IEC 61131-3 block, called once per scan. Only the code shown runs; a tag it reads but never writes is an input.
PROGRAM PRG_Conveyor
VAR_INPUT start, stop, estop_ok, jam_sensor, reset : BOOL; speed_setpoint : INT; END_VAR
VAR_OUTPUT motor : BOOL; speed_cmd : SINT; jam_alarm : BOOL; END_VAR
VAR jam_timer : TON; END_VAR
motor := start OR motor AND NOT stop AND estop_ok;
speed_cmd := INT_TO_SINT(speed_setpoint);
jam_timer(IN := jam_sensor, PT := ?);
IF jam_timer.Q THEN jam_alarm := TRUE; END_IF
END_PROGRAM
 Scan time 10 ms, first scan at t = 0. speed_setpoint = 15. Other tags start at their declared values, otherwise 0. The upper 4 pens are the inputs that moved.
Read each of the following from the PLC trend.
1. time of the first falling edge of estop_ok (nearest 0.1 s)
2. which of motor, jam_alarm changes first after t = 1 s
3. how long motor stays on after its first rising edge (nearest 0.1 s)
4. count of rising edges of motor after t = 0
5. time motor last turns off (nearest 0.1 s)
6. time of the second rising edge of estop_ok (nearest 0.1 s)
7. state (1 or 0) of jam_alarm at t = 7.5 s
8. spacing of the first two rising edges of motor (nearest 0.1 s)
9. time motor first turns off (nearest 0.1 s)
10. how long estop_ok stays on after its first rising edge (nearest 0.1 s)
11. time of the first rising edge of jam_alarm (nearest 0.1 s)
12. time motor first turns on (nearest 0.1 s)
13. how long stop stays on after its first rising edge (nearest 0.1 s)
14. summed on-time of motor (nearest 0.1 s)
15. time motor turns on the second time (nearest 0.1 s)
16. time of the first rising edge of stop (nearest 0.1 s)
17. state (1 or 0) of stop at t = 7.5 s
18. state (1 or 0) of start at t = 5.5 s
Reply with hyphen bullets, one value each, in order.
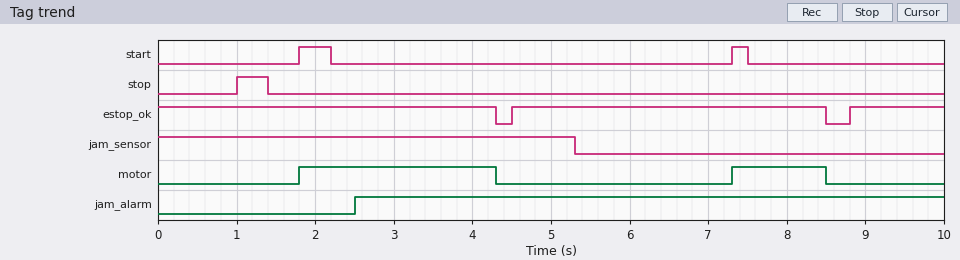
- 4.3 s
- motor
- 2.5 s
- 2
- 8.5 s
- 8.8 s
- 1
- 5.5 s
- 4.3 s
- 4.0 s
- 2.5 s
- 1.8 s
- 0.4 s
- 3.7 s
- 7.3 s
- 1.0 s
- 0
- 0
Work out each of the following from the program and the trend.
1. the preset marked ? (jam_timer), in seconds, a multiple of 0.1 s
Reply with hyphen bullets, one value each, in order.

- 2.5 s
